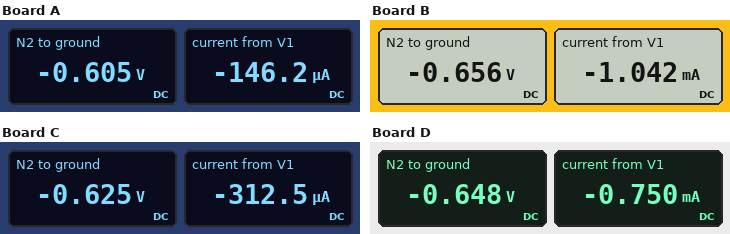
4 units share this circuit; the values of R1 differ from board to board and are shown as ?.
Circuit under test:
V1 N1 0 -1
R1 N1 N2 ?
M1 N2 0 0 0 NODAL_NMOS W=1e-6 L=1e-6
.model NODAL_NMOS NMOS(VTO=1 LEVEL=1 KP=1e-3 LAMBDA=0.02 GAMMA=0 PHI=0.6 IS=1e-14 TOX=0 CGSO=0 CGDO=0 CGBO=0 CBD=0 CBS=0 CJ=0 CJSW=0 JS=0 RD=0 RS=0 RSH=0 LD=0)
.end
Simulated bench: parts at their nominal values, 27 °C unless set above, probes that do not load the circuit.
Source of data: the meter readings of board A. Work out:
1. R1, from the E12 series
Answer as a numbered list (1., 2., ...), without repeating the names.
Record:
1. 2.7 kΩ
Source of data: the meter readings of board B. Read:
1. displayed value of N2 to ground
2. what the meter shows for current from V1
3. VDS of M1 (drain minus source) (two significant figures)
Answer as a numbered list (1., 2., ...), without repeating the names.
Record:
1. -0.656 V
2. -1.042 mA
3. -660 mV
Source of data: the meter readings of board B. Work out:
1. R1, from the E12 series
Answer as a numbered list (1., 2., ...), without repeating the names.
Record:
1. 330 Ω
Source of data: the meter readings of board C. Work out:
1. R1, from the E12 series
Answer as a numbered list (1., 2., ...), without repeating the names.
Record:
1. 1.2 kΩ
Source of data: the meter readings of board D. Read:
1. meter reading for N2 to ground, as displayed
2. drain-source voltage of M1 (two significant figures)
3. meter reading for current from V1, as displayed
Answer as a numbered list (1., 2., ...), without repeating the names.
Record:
1. -0.648 V
2. -650 mV
3. -0.750 mA
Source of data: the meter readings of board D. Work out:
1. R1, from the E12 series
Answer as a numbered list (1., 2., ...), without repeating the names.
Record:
1. 470 Ω
